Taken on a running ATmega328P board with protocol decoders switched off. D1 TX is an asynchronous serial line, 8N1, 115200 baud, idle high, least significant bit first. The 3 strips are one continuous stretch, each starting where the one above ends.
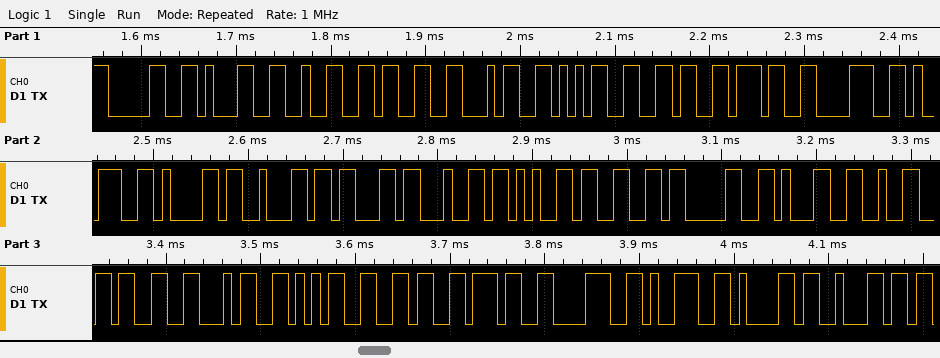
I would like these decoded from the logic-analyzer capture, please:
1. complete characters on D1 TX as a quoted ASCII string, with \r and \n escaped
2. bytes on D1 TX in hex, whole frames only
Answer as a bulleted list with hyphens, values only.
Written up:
- "0123456789abcdef0123456789ab"
- 30 31 32 33 34 35 36 37 38 39 61 62 63 64 65 66 30 31 32 33 34 35 36 37 38 39 61 62
